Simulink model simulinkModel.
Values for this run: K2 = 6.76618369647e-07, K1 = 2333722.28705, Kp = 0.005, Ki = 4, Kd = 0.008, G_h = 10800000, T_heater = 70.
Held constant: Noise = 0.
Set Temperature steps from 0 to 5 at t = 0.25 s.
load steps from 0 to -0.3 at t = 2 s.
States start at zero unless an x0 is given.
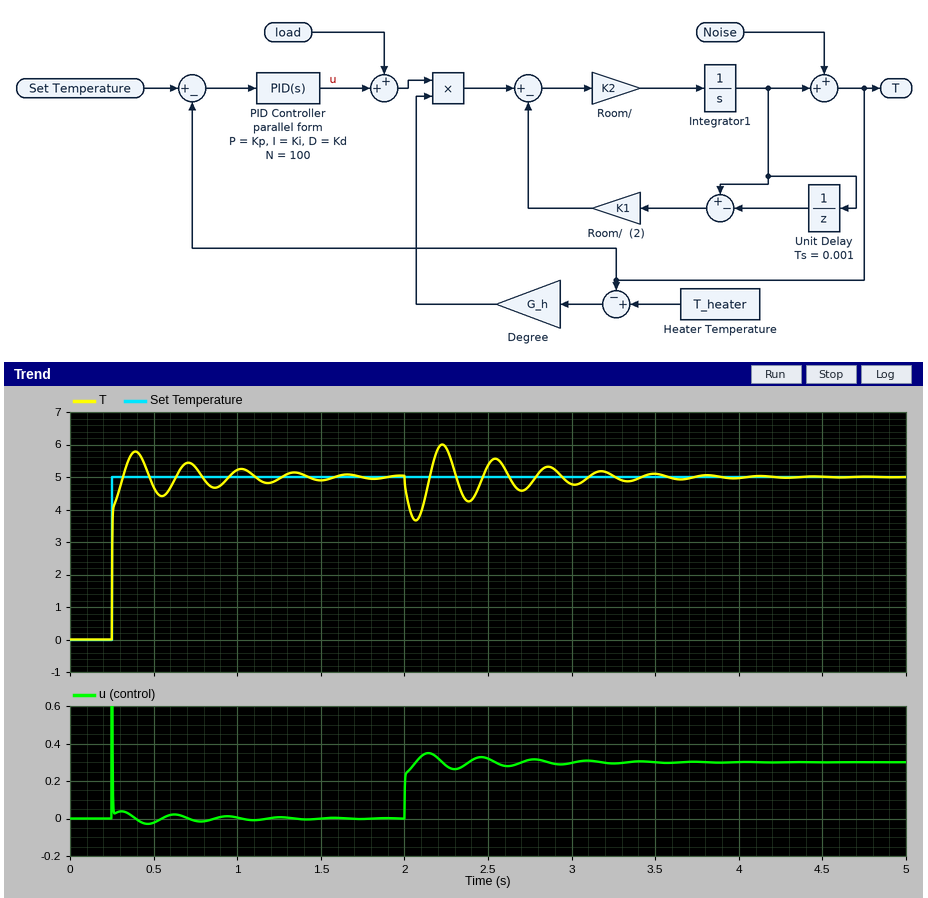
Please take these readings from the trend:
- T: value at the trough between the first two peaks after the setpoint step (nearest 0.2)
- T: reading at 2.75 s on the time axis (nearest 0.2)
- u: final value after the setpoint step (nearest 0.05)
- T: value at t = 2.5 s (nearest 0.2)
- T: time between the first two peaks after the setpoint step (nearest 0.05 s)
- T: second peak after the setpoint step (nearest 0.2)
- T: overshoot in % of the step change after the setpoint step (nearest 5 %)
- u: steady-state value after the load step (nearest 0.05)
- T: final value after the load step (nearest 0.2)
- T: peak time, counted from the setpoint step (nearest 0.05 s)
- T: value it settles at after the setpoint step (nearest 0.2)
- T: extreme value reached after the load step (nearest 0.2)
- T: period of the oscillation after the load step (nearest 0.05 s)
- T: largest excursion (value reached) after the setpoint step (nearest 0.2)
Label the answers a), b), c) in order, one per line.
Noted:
a) 4.4
b) 4.8
c) 0.00
d) 5.4
e) 0.30 s
f) 5.4
g) 15 %
h) 0.30
i) 5.0
j) 0.15 s
k) 5.0
l) 3.6
m) 0.30 s
n) 5.8
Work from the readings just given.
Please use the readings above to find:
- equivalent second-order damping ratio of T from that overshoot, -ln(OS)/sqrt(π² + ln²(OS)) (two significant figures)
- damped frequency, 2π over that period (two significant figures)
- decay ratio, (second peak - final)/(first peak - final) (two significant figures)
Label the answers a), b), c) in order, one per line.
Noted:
a) 0.52
b) 21 rad/s
c) 0.50
